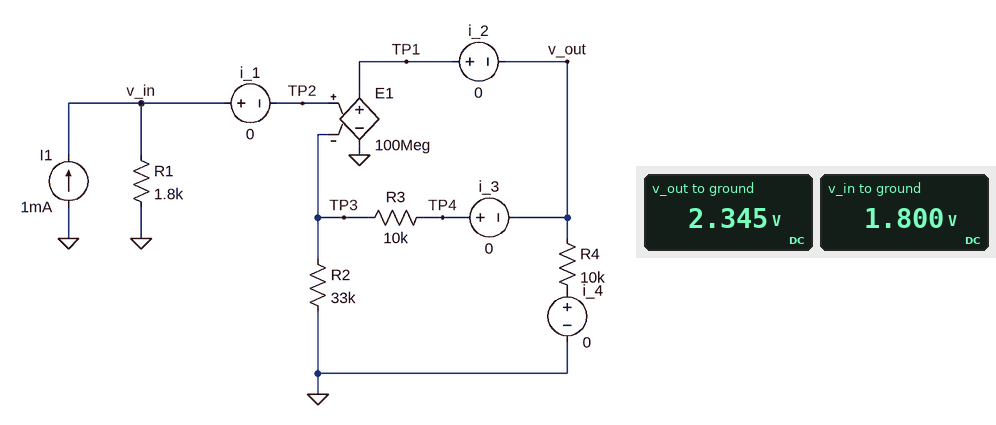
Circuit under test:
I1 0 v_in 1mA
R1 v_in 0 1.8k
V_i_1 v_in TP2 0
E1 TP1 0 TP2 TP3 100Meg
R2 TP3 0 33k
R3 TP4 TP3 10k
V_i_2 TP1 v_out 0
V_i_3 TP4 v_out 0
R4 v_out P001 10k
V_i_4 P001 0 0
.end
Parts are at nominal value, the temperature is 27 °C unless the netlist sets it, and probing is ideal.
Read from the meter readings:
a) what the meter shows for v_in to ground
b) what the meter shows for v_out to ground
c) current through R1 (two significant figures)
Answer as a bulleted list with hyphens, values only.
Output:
- 1.800 V
- 2.345 V
- 1.0 mA
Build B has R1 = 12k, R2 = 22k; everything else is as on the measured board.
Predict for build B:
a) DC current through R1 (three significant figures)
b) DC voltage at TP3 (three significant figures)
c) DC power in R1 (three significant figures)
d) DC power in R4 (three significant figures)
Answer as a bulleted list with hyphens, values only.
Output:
- 1.00 mA
- 12.0 V
- 12.0 mW
- 30.5 mW
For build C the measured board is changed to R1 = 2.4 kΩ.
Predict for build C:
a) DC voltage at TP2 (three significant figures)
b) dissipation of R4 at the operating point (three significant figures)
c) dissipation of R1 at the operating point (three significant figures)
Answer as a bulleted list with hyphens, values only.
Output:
- 2.40 V
- 978 µW
- 2.40 mW
